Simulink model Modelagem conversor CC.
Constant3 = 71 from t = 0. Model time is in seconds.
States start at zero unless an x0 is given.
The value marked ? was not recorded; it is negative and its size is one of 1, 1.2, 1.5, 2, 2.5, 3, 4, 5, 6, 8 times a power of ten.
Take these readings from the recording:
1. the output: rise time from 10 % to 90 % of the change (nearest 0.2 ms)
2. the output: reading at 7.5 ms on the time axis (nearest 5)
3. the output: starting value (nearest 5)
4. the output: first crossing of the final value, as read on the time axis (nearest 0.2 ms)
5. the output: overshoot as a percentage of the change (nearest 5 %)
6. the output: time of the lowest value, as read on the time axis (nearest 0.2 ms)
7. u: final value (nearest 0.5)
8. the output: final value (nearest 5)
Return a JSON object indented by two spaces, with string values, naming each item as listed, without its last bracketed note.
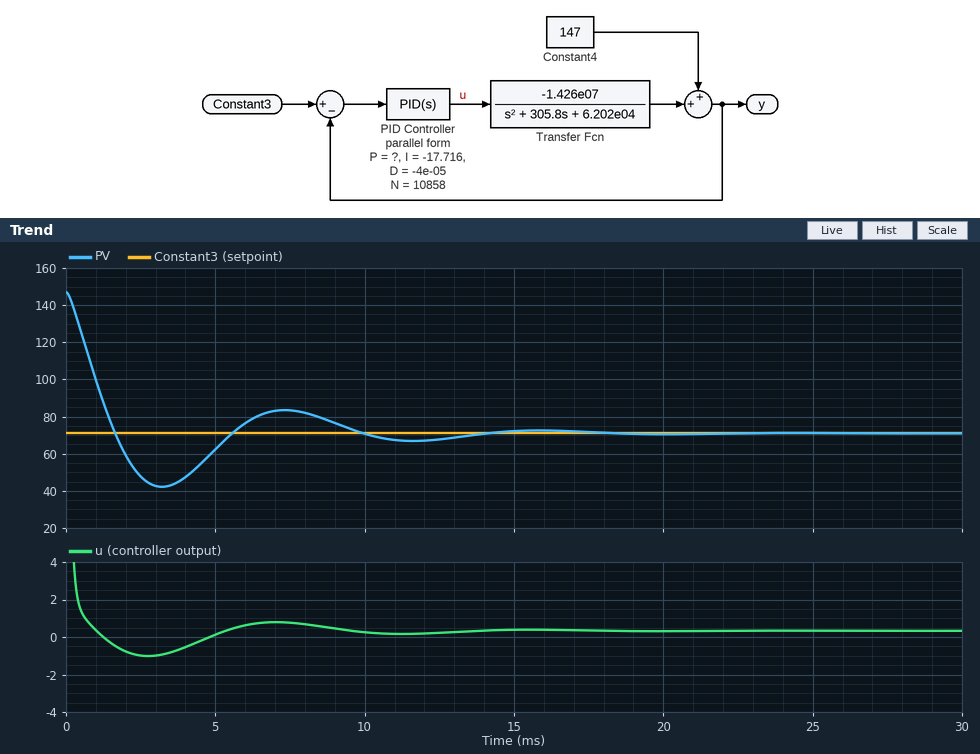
{
  "the output: rise time from 10 % to 90 % of the change": "1.2 ms",
  "the output: reading at 7.5 ms on the time axis": "85",
  "the output: starting value": "145",
  "the output: first crossing of the final value, as read on the time axis": "1.6 ms",
  "the output: overshoot as a percentage of the change": "40 %",
  "the output: time of the lowest value, as read on the time axis": "3.2 ms",
  "u: final value": "0.5",
  "the output: final value": "70"
}
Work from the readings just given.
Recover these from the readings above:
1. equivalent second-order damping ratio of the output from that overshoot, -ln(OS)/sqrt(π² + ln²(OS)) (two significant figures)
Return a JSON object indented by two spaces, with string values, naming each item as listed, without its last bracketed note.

{
  "equivalent second-order damping ratio of the output from that overshoot, -ln(OS)/sqrt(π² + ln²(OS))": "0.28"
}
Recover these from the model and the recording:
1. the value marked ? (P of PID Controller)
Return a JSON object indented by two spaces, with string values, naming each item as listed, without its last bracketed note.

{
  "the value marked ?": "-0.05"
}
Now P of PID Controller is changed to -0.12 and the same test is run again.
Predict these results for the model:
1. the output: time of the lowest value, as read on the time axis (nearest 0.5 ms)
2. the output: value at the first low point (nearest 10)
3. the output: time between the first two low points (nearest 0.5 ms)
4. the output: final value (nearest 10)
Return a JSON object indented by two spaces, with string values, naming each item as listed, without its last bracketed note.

{
  "the output: time of the lowest value, as read on the time axis": "2.0 ms",
  "the output: value at the first low point": "40",
  "the output: time between the first two low points": "5.0 ms",
  "the output: final value": "70"
}
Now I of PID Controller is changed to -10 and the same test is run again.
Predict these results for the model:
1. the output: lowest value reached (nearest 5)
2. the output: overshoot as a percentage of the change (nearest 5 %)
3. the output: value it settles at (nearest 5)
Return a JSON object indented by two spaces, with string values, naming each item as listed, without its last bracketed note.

{
  "the output: lowest value reached": "50",
  "the output: overshoot as a percentage of the change": "30 %",
  "the output: value it settles at": "70"
}
